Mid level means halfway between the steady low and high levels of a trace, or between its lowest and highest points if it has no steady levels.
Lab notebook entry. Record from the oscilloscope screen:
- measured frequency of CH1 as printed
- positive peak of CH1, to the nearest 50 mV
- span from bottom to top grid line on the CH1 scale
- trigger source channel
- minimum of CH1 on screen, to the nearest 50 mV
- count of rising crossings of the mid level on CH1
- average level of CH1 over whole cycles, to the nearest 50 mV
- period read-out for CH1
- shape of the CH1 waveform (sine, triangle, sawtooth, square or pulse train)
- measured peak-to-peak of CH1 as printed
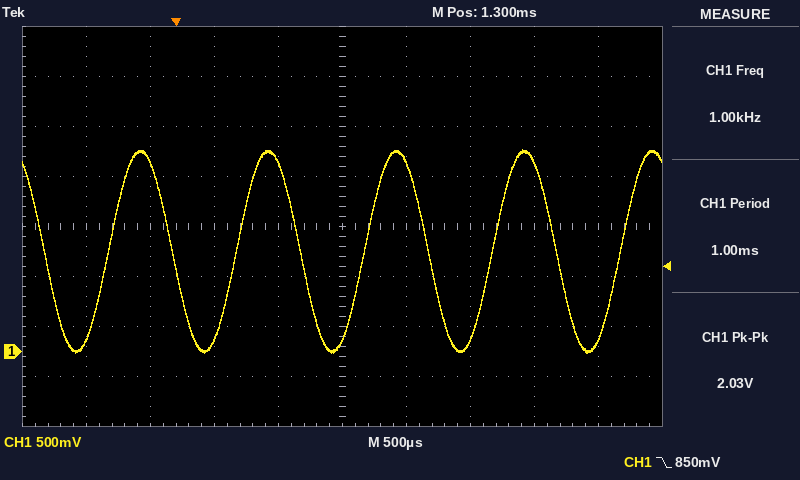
1.00 kHz
2.00 V
4 V
CH1
0 mV
5
1.00 V
1.00 ms
sine
2.03 V
